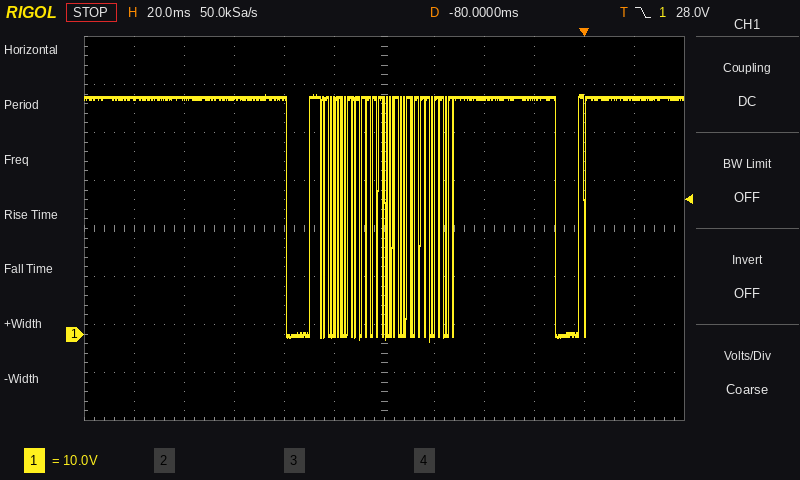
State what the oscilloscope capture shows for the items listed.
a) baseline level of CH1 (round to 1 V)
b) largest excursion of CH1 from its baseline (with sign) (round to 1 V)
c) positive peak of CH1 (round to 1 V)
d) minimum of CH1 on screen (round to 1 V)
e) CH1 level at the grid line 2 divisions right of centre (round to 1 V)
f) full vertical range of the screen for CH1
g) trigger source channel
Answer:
49 V
-51 V
50 V
-2 V
49 V
80 V
CH1
